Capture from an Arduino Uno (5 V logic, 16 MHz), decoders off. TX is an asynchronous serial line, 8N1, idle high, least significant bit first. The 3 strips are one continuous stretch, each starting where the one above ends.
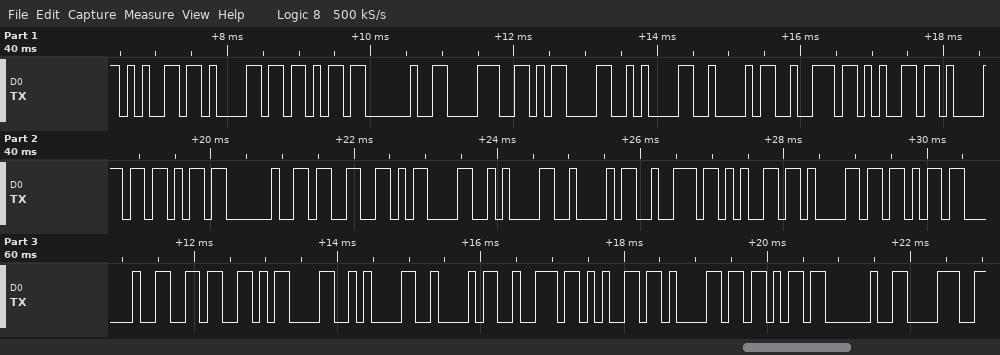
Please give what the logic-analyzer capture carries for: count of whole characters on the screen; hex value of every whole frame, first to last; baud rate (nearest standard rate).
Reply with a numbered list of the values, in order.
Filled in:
1. 32
2. 65 61 6B 20 38 0D 0A 42 72 65 61 6B 20 33 0D 0A 42 72 65 61 6B 20 36 0D 0A 42 72 65 61 6B 20 38
3. 9600 baud
